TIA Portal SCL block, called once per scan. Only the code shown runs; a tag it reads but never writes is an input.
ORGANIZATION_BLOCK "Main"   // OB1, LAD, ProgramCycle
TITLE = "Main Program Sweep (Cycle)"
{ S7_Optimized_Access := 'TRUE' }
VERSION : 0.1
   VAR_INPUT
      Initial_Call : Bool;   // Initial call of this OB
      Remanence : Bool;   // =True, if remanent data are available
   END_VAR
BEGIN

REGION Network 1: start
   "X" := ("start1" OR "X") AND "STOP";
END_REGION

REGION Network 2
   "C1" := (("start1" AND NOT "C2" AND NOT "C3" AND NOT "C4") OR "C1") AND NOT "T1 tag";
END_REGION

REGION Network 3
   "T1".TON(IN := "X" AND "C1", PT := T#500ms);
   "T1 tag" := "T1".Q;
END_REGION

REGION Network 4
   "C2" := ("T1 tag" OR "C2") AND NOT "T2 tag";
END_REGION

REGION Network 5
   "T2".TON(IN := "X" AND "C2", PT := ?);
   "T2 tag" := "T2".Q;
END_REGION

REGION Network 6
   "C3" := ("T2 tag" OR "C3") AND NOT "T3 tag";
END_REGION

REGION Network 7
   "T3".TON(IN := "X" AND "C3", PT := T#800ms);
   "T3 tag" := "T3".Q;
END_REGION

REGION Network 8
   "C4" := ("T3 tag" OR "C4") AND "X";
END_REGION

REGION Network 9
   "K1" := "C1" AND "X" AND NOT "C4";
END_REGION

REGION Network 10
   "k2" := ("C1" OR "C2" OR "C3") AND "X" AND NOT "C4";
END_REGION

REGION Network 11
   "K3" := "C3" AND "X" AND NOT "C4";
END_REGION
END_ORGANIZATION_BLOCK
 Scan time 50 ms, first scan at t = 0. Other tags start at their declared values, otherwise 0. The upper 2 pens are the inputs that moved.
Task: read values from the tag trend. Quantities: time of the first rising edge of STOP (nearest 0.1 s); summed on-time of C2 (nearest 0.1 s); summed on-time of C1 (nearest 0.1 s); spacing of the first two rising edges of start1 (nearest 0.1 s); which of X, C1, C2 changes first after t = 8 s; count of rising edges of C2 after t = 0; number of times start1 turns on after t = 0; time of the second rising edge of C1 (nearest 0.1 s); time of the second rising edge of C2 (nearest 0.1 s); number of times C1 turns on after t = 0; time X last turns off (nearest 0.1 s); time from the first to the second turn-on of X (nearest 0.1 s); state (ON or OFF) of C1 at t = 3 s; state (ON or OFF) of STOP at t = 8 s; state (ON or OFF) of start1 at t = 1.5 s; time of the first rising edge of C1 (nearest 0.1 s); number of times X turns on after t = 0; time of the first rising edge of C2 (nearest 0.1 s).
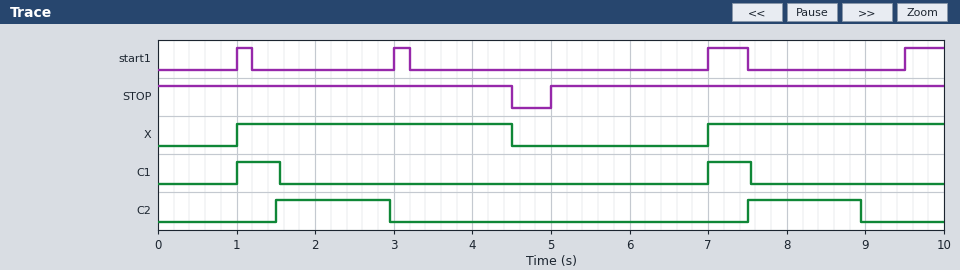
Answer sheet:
5.0 s
2.9 s
1.1 s
2.0 s
C2
2
4
7.0 s
7.5 s
2
4.5 s
6.0 s
OFF
ON
OFF
1.0 s
2
1.5 s
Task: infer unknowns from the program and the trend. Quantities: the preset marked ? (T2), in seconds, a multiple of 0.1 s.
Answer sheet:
1.4 s
